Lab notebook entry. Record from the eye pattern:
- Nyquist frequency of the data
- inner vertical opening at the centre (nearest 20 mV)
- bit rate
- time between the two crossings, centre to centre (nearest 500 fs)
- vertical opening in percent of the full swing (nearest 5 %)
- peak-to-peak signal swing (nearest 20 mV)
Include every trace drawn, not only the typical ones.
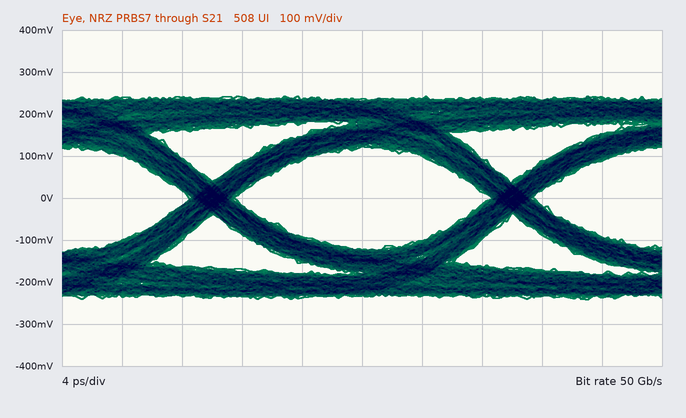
25 GHz
240 mV
50 Gb/s
20.0 ps
50 %
480 mV
